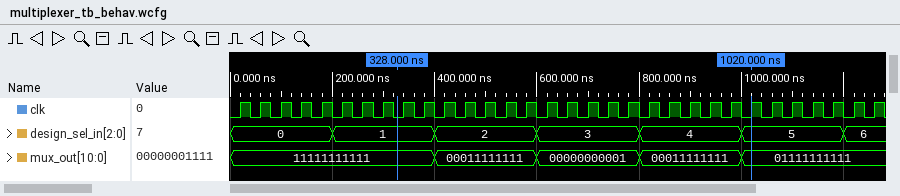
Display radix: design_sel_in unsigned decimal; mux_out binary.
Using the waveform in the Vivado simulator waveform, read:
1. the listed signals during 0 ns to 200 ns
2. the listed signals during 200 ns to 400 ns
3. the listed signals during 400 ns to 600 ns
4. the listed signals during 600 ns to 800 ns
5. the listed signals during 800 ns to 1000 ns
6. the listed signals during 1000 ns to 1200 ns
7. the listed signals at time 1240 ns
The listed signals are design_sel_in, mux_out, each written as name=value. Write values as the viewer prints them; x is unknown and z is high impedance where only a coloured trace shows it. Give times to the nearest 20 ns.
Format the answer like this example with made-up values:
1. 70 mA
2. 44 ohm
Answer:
1. design_sel_in=0, mux_out=11111111111
2. design_sel_in=1, mux_out=11111111111
3. design_sel_in=2, mux_out=00011111111
4. design_sel_in=3, mux_out=00000000001
5. design_sel_in=4, mux_out=00011111111
6. design_sel_in=5, mux_out=01111111111
7. design_sel_in=6, mux_out=01111111111
